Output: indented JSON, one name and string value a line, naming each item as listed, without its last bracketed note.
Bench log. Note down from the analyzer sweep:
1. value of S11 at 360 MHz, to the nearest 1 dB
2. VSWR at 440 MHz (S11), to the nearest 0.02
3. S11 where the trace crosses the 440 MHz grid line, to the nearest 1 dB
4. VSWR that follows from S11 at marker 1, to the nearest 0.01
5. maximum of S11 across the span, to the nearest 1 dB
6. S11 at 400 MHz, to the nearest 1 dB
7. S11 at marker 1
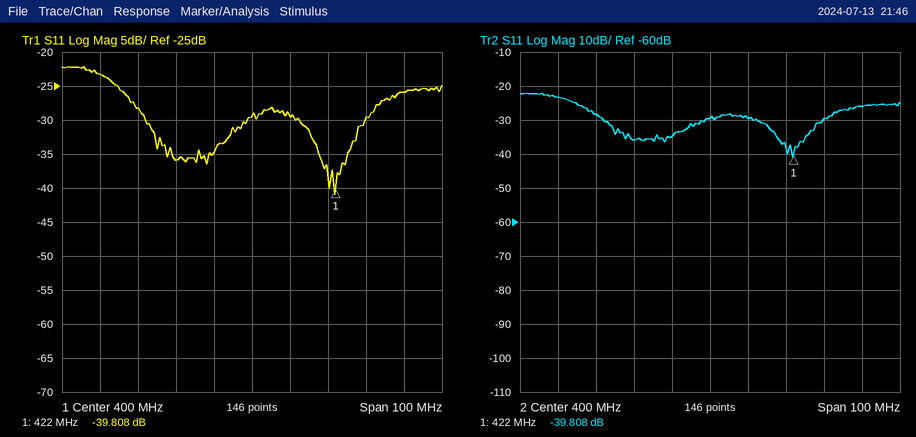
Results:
{
  "value of S11 at 360 MHz, to the nearest 1 dB": "-23 dB",
  "VSWR at 440 MHz (S11), to the nearest 0.02": "1.10",
  "S11 where the trace crosses the 440 MHz grid line, to the nearest 1 dB": "-26 dB",
  "VSWR that follows from S11 at marker 1, to the nearest 0.01": "1.02",
  "maximum of S11 across the span, to the nearest 1 dB": "-22 dB",
  "S11 at 400 MHz, to the nearest 1 dB": "-29 dB",
  "S11 at marker 1": "-39.808 dB"
}
